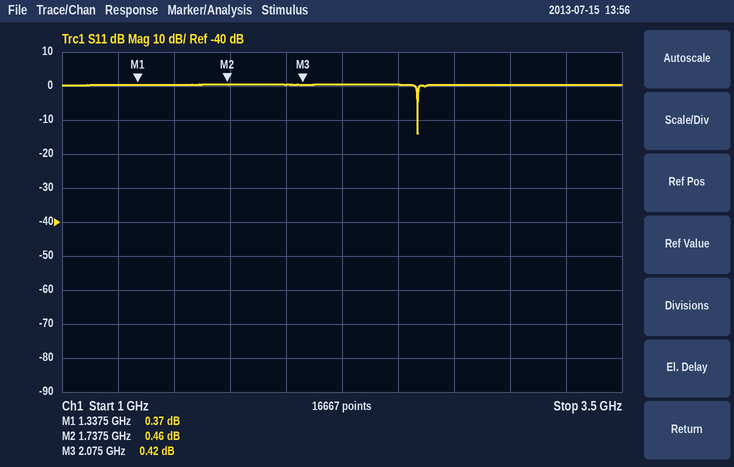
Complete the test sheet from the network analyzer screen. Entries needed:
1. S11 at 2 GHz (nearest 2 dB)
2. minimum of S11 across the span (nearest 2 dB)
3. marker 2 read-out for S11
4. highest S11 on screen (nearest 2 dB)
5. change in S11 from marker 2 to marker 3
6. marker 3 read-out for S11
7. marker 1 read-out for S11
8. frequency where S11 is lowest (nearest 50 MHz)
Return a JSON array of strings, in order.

["0 dB", "-14 dB", "0.46 dB", "0 dB", "-0.04 dB", "0.42 dB", "0.37 dB", "2.60 GHz"]
